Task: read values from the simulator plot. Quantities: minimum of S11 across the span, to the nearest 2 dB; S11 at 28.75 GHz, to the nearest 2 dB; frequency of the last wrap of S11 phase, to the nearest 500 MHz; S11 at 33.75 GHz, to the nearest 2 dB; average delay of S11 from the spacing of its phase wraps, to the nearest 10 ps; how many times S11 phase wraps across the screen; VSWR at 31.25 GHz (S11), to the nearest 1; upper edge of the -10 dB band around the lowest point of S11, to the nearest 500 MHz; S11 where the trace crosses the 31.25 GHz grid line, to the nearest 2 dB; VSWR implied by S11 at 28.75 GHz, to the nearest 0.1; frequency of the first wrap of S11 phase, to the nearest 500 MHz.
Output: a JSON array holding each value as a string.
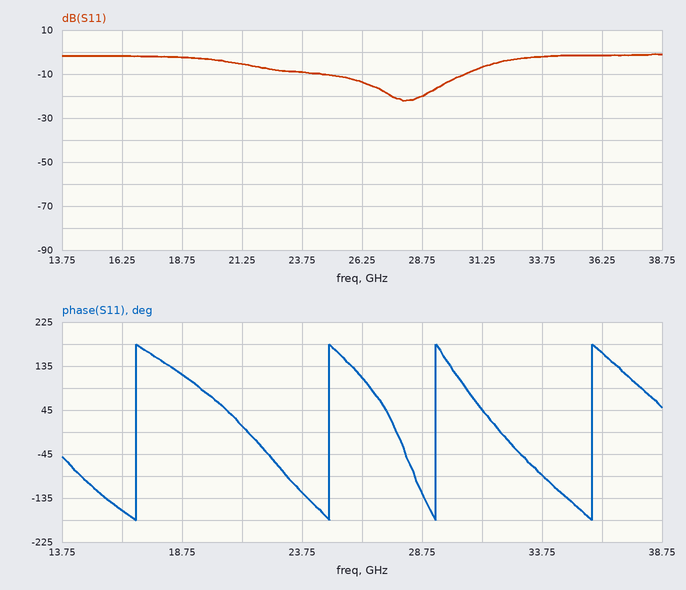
["-22 dB", "-20 dB", "36.0 GHz", "-2 dB", "160 ps", "4", "3", "30.5 GHz", "-6 dB", "1.2", "17.0 GHz"]
